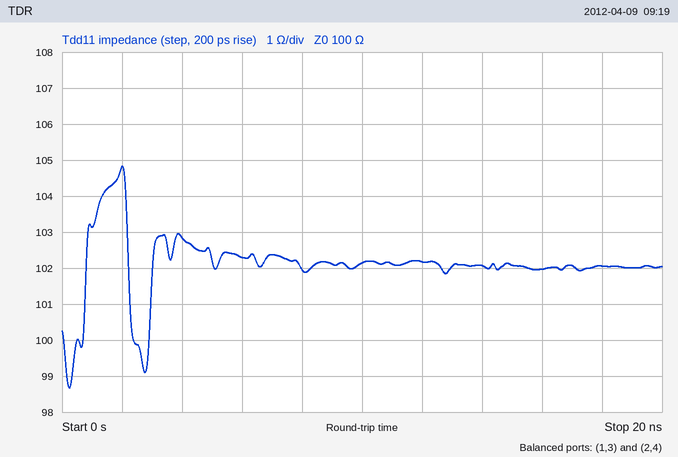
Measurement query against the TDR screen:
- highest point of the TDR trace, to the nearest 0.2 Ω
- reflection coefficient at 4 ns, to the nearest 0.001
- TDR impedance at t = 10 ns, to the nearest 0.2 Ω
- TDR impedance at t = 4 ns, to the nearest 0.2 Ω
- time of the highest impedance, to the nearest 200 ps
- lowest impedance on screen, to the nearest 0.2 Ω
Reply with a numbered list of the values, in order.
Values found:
1. 104.8 Ω
2. +0.014
3. 102.2 Ω
4. 102.8 Ω
5. 2.0 ns
6. 98.6 Ω
